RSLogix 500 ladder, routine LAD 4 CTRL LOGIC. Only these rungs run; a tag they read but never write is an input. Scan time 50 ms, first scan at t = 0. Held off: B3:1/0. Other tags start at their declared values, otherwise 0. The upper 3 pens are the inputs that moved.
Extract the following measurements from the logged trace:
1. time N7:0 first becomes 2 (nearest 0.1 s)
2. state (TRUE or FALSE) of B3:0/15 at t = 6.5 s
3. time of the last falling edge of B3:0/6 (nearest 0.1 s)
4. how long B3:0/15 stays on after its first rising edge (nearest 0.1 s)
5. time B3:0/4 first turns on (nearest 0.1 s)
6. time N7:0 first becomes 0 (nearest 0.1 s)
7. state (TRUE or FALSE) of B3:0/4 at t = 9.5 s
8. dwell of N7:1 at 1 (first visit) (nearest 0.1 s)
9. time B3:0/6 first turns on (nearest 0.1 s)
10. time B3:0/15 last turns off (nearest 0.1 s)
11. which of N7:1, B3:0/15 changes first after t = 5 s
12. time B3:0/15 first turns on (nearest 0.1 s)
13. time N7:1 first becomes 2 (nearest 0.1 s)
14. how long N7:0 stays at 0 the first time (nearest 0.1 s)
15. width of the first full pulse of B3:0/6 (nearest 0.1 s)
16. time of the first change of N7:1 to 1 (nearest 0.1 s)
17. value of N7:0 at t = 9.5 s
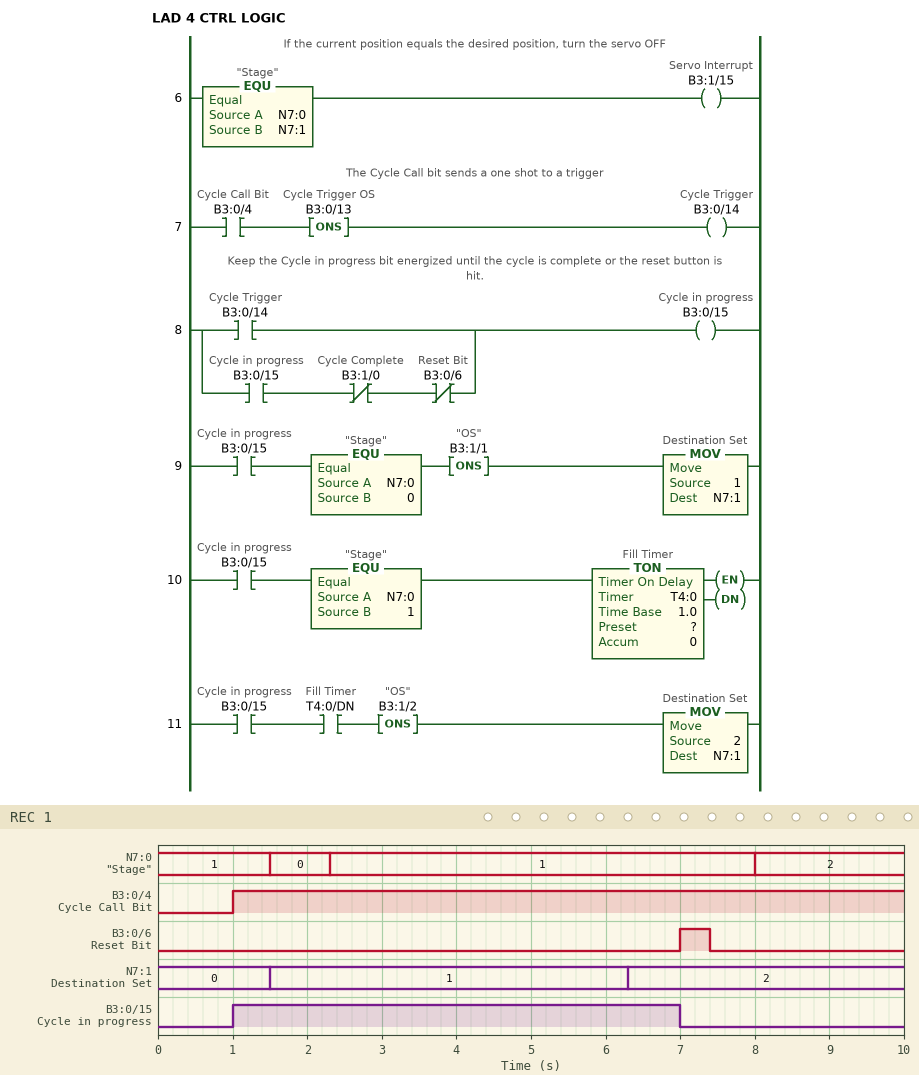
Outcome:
8.0 s
TRUE
7.4 s
6.0 s
1.0 s
1.5 s
TRUE
4.8 s
7.0 s
7.0 s
N7:1
1.0 s
6.3 s
0.8 s
0.4 s
1.5 s
2
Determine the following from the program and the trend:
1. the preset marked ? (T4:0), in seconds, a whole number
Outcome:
4 s
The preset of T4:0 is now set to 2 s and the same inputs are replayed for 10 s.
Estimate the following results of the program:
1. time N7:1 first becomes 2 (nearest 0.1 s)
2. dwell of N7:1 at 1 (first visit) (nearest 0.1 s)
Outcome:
4.3 s
2.8 s
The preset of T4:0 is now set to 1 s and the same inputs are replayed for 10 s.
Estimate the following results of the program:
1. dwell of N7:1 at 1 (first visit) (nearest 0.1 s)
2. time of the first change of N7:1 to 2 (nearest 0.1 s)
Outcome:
1.8 s
3.3 s
